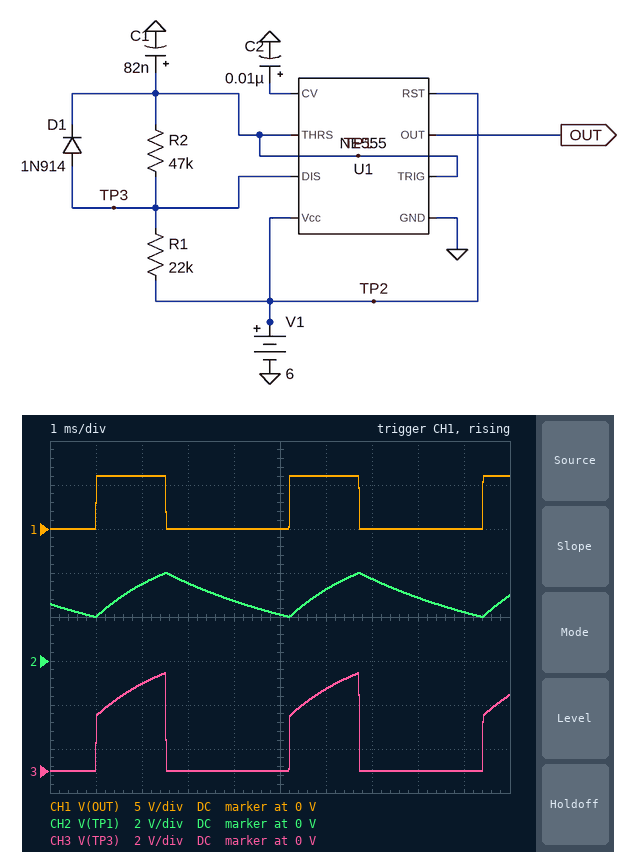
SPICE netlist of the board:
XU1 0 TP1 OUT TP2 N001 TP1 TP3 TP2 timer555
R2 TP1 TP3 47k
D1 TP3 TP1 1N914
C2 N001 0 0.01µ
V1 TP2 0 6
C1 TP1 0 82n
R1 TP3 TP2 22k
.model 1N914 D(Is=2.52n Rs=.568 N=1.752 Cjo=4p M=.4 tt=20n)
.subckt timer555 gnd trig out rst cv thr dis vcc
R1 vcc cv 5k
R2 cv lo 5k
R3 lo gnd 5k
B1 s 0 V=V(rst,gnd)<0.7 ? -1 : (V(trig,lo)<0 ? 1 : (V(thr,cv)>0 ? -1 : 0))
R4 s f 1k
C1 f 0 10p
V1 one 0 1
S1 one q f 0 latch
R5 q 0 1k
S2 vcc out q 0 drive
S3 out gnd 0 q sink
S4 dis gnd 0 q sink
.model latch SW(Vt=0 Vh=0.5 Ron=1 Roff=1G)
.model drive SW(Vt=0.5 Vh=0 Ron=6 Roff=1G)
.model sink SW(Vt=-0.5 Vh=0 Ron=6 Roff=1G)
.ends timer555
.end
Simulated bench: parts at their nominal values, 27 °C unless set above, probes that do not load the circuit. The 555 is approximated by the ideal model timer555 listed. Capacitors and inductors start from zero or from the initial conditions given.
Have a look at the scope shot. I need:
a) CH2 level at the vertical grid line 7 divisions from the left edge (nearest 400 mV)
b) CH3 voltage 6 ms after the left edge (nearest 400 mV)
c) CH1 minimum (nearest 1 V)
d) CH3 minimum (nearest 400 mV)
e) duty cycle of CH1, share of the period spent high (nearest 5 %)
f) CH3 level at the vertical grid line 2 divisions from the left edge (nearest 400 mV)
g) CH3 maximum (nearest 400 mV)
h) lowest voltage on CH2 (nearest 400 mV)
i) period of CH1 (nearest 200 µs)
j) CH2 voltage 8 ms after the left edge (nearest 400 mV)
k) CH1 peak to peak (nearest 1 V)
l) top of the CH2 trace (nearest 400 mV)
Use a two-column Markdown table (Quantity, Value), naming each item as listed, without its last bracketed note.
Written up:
| Quantity | Value |
|---|---|
| CH2 level at the vertical grid line 7 divisions from the left edge | 3.6 V |
| CH3 voltage 6 ms after the left edge | 3.6 V |
| CH1 minimum | 0 V |
| CH3 minimum | 0 V |
| duty cycle of CH1, share of the period spent high | 35 % |
| CH3 level at the vertical grid line 2 divisions from the left edge | 4.0 V |
| CH3 maximum | 4.4 V |
| lowest voltage on CH2 | 2.0 V |
| period of CH1 | 4.2 ms |
| CH2 voltage 8 ms after the left edge | 2.8 V |
| CH1 peak to peak | 6 V |
| top of the CH2 trace | 4.0 V |
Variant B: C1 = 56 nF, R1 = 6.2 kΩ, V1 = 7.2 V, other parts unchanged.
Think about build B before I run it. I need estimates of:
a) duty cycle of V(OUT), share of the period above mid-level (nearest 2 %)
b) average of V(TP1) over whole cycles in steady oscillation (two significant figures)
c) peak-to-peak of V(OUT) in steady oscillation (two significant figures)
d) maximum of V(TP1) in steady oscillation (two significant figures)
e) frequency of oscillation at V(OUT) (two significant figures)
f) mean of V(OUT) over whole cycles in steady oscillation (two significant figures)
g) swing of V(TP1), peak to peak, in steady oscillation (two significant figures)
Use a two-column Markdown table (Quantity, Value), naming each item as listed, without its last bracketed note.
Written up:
| Quantity | Value |
|---|---|
| duty cycle of V(OUT), share of the period above mid-level | 14 % |
| average of V(TP1) over whole cycles in steady oscillation | 3.5 V |
| peak-to-peak of V(OUT) in steady oscillation | 7.2 V |
| maximum of V(TP1) in steady oscillation | 4.8 V |
| frequency of oscillation at V(OUT) | 470 Hz |
| mean of V(OUT) over whole cycles in steady oscillation | 980 mV |
| swing of V(TP1), peak to peak, in steady oscillation | 2.4 V |
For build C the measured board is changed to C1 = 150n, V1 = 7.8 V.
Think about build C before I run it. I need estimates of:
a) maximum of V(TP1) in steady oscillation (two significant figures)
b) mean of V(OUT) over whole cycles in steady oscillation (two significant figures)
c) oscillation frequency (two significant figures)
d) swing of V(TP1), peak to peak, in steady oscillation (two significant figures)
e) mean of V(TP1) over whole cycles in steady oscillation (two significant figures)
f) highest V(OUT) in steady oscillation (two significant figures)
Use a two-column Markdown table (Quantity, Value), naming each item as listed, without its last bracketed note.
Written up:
| Quantity | Value |
|---|---|
| maximum of V(TP1) in steady oscillation | 5.2 V |
| mean of V(OUT) over whole cycles in steady oscillation | 2.7 V |
| oscillation frequency | 130 Hz |
| swing of V(TP1), peak to peak, in steady oscillation | 2.6 V |
| mean of V(TP1) over whole cycles in steady oscillation | 3.9 V |
| highest V(OUT) in steady oscillation | 7.8 V |
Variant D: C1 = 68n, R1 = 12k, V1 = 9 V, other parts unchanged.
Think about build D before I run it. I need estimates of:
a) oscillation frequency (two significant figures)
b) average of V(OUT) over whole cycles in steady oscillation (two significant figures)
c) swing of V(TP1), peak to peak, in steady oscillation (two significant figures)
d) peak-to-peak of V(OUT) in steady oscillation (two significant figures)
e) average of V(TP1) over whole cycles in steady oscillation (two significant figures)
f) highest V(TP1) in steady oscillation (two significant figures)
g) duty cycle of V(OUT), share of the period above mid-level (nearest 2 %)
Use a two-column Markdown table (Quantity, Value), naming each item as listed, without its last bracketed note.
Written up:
| Quantity | Value |
|---|---|
| oscillation frequency | 350 Hz |
| average of V(OUT) over whole cycles in steady oscillation | 2.0 V |
| swing of V(TP1), peak to peak, in steady oscillation | 3.0 V |
| peak-to-peak of V(OUT) in steady oscillation | 9.0 V |
| average of V(TP1) over whole cycles in steady oscillation | 4.4 V |
| highest V(TP1) in steady oscillation | 6.0 V |
| duty cycle of V(OUT), share of the period above mid-level | 22 % |
